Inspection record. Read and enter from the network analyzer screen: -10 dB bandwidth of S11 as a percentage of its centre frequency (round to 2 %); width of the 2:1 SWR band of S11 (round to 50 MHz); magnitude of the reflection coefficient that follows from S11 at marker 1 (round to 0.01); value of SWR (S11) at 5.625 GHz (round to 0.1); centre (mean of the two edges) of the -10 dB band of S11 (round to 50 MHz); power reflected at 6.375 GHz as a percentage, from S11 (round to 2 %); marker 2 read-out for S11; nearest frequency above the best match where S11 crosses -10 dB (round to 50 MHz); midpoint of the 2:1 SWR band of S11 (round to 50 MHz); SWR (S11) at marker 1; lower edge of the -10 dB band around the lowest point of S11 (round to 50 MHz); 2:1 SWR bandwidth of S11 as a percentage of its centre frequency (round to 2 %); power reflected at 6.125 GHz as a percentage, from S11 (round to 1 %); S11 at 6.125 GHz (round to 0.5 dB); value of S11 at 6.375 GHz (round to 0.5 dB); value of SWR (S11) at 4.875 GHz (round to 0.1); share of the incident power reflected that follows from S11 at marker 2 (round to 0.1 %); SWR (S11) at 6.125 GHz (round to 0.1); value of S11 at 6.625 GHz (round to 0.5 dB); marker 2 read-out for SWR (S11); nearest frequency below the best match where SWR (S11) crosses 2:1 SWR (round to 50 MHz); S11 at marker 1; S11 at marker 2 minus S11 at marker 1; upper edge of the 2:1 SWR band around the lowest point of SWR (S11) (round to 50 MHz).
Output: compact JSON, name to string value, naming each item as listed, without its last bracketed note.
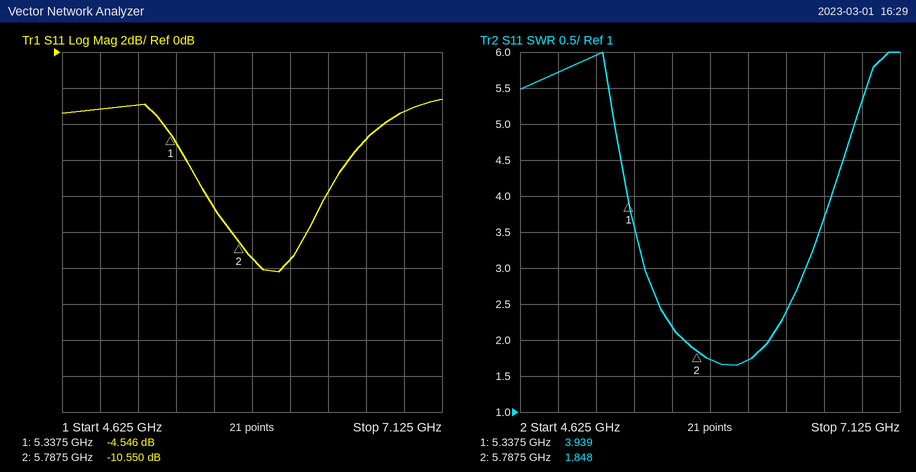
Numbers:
{"-10 dB bandwidth of S11 as a percentage of its centre frequency": "8 %", "width of the 2:1 SWR band of S11": "550 MHz", "magnitude of the reflection coefficient that follows from S11 at marker 1": "0.59", "value of SWR (S11) at 5.625 GHz": "2.2", "centre (mean of the two edges) of the -10 dB band of S11": "6.00 GHz", "power reflected at 6.375 GHz as a percentage, from S11": "16 %", "marker 2 read-out for S11": "-10.550 dB", "nearest frequency above the best match where S11 crosses -10 dB": "6.25 GHz", "midpoint of the 2:1 SWR band of S11": "6.00 GHz", "SWR (S11) at marker 1": "3.939", "lower edge of the -10 dB band around the lowest point of S11": "5.75 GHz", "2:1 SWR bandwidth of S11 as a percentage of its centre frequency": "10 %", "power reflected at 6.125 GHz as a percentage, from S11": "7 %", "S11 at 6.125 GHz": "-11.5 dB", "value of S11 at 6.375 GHz": "-8.0 dB", "value of SWR (S11) at 4.875 GHz": "5.7", "share of the incident power reflected that follows from S11 at marker 2": "8.8 %", "SWR (S11) at 6.125 GHz": "1.7", "value of S11 at 6.625 GHz": "-5.0 dB", "marker 2 read-out for SWR": "1.848", "nearest frequency below the best match where SWR (S11) crosses 2:1 SWR": "5.70 GHz", "S11 at marker 1": "-4.546 dB", "S11 at marker 2 minus S11 at marker 1": "-6.004 dB", "upper edge of the 2:1 SWR band around the lowest point of SWR (S11)": "6.25 GHz"}
